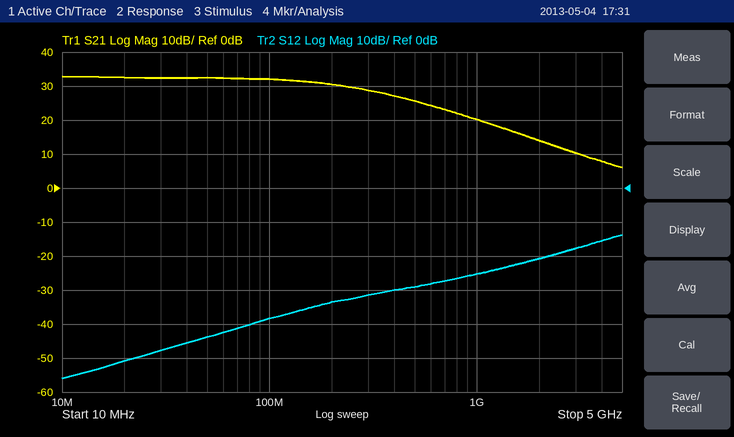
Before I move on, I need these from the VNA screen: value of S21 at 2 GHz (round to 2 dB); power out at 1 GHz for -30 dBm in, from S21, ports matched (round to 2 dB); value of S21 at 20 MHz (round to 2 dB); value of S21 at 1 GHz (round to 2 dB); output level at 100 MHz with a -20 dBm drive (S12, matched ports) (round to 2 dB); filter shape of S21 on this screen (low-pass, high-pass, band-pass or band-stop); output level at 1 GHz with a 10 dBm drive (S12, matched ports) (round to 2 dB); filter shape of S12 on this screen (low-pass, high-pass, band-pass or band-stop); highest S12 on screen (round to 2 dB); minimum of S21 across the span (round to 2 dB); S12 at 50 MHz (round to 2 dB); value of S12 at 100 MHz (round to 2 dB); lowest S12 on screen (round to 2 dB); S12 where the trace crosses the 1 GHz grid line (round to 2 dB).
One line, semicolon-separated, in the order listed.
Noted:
14 dB; -10 dBm; 32 dB; 20 dB; -58 dBm; low-pass; -16 dBm; high-pass; -14 dB; 6 dB; -44 dB; -38 dB; -56 dB; -26 dB
